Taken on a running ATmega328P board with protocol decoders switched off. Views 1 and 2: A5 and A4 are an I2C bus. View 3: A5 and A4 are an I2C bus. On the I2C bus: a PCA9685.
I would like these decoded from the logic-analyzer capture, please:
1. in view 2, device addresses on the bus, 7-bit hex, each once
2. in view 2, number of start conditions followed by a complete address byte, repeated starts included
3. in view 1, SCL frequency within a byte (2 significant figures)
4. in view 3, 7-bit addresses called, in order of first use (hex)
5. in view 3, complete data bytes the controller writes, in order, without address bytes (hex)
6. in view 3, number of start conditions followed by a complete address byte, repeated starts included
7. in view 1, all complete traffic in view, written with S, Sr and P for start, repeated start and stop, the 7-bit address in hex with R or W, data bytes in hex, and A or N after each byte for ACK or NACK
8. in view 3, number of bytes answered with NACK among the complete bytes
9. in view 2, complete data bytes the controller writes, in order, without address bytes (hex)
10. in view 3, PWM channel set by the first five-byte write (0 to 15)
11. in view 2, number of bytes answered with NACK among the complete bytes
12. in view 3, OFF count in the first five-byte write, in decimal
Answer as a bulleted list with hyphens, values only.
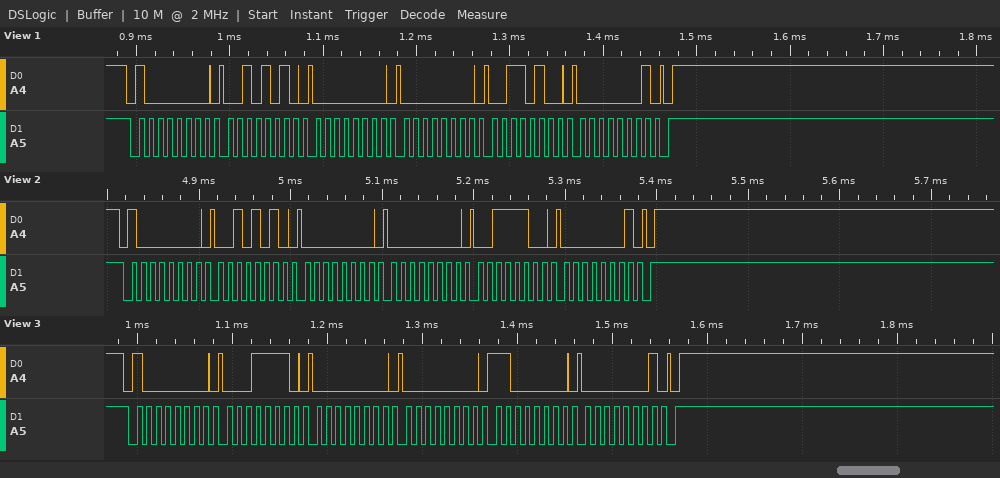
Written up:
- 0x40
- 1
- 100 kHz
- 0x40
- 1E 00 00 C0 01
- 1
- S 40W A 2A A 00 A 00 A 34 A 01 A P
- 0
- 2A 00 00 3C 01
- 6
- 0
- 448
